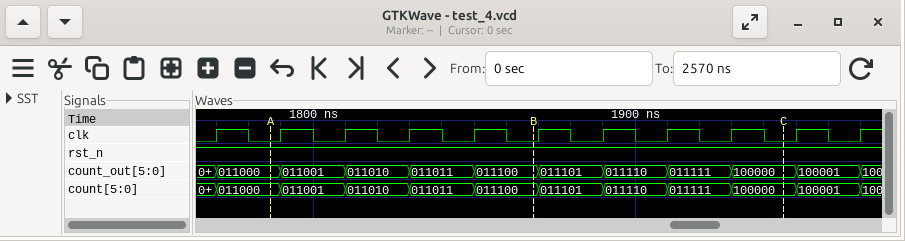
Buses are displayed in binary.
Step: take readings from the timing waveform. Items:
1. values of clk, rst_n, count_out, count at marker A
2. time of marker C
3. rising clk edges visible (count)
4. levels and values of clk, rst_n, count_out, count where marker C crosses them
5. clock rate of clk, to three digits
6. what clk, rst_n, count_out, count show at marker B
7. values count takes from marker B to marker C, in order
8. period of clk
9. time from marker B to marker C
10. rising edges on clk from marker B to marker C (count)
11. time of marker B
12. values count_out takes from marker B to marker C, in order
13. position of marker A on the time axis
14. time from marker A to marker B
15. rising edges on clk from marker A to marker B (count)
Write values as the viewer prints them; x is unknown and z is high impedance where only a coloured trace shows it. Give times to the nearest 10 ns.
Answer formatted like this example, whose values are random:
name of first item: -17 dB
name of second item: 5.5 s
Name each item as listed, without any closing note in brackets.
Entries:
values of clk, rst_n, count_out, count at marker A: clk=0, rst_n=1, count_out=011000, count=011000
time of marker C: 1950 ns
rising clk edges visible: 11
levels and values of clk, rst_n, count_out, count where marker C crosses them: clk=0, rst_n=1, count_out=100000, count=100000
clock rate of clk, to three digits: 50.0 MHz
what clk, rst_n, count_out, count show at marker B: clk=0, rst_n=1, count_out=011100, count=011100
values count takes from marker B to marker C, in order: 011100, 011101, 011110, 011111, 100000
period of clk: 20 ns
time from marker B to marker C: 80 ns
rising edges on clk from marker B to marker C: 4
time of marker B: 1870 ns
values count_out takes from marker B to marker C, in order: 011100, 011101, 011110, 011111, 100000
position of marker A on the time axis: 1790 ns
time from marker A to marker B: 80 ns
rising edges on clk from marker A to marker B: 4
